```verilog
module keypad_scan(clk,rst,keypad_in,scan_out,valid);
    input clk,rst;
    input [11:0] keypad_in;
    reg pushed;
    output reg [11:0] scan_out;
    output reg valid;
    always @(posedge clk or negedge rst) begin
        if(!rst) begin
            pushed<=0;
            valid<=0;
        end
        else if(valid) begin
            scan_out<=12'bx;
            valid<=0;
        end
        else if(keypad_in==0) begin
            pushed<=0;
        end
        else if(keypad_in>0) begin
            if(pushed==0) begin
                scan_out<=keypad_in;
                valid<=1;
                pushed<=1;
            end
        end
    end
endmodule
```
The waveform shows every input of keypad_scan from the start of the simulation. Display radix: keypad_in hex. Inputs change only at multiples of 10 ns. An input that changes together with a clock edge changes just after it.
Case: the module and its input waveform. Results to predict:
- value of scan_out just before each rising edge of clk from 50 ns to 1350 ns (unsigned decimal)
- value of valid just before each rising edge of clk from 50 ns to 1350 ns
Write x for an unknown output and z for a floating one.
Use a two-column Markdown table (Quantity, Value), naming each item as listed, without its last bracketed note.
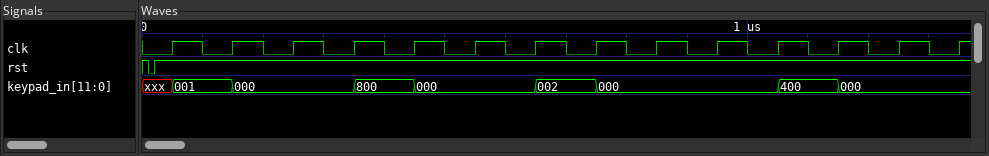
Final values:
| Quantity | Value |
|---|---|
| value of scan_out just before each rising edge of clk from 50 ns to 1350 ns | x, x, 1, x, x, 2048, x, x, 2, x, x, x, 1024, x |
| value of valid just before each rising edge of clk from 50 ns to 1350 ns | 0 0 1 0 0 1 0 0 1 0 0 0 1 0 |
